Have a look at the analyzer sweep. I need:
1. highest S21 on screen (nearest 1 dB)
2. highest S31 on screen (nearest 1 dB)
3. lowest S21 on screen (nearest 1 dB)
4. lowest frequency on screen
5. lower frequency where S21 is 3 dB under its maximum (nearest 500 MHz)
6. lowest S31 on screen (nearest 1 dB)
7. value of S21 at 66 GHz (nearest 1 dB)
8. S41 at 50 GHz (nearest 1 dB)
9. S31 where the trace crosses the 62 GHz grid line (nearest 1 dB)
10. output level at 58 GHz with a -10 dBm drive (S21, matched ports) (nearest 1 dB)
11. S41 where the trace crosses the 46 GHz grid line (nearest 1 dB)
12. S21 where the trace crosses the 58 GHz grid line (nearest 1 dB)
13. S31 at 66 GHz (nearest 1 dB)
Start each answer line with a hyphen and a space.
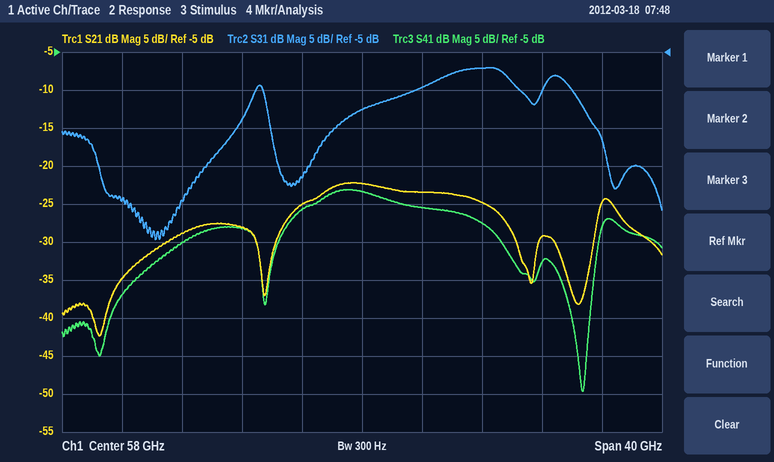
- -22 dB
- -7 dB
- -42 dB
- 38 GHz
- 54.0 GHz
- -30 dB
- -25 dB
- -28 dB
- -10 dB
- -32 dBm
- -30 dB
- -22 dB
- -7 dB
